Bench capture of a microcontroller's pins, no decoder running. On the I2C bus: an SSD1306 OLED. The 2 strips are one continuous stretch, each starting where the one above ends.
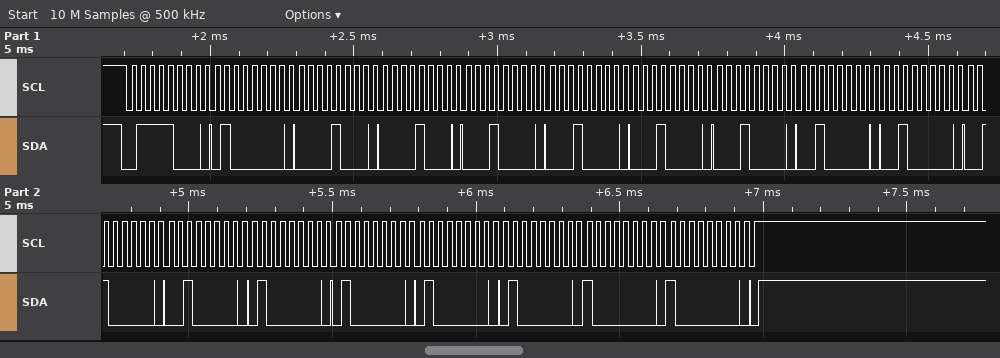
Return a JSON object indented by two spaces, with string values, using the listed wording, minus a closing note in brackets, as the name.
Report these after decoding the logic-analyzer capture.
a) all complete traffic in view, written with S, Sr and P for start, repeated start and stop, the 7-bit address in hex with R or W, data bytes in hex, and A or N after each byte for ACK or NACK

{
  "all complete traffic in view, written with S, Sr and P for start, repeated start and stop, the 7-bit address in hex with R or W, data bytes in hex, and A or N after each byte for ACK or NACK": "S 3CW A 40 A 08 A 08 A 10 A 10 A 10 A 10 A 20 A 20 A 20 A 20 A 40 A 40 A 40 A 40 A 80 A 80 A P"
}
